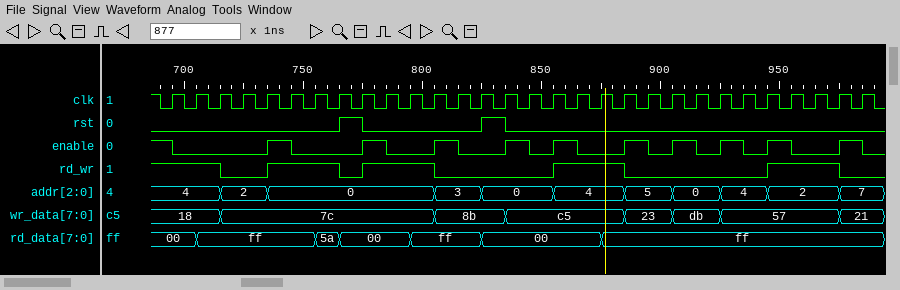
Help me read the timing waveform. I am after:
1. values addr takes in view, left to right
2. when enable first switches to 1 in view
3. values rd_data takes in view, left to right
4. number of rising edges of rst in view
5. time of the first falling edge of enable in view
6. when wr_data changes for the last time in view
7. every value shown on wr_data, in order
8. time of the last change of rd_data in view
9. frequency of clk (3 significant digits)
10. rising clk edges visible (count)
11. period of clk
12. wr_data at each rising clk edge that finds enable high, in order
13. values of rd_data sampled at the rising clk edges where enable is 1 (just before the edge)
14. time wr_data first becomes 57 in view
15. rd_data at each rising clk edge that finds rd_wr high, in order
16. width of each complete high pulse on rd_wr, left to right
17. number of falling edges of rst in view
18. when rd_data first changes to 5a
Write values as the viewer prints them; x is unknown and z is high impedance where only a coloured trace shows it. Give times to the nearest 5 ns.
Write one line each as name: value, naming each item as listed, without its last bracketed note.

values addr takes in view, left to right: 4, 2, 0, 3, 0, 4, 5, 0, 4, 2, 7
when enable first switches to 1 in view: 735 ns
values rd_data takes in view, left to right: 00, ff, 5a, 00, ff, 00, ff
number of rising edges of rst in view: 2
time of the first falling edge of enable in view: 695 ns
when wr_data changes for the last time in view: 975 ns
every value shown on wr_data, in order: 18, 7c, 8b, c5, 23, db, 57, 21
time of the last change of rd_data in view: 875 ns
frequency of clk: 100 MHz
rising clk edges visible: 30
period of clk: 10 ns
wr_data at each rising clk edge that finds enable high, in order: 18, 7c, 7c, 8b, c5, c5, 23, db, 57, 57, 21
values of rd_data sampled at the rising clk edges where enable is 1: 00, ff, 00, ff, 00, 00, ff, ff, ff, ff, ff
time wr_data first becomes 57 in view: 925 ns
rd_data at each rising clk edge that finds rd_wr high, in order: 00, 00, ff, ff, ff, 5a, 00, 00, ff, 00, 00, ff, ff, ff, ff
width of each complete high pulse on rd_wr, left to right: 30 ns, 30 ns, 30 ns, 30 ns
number of falling edges of rst in view: 2
when rd_data first changes to 5a: 755 ns
